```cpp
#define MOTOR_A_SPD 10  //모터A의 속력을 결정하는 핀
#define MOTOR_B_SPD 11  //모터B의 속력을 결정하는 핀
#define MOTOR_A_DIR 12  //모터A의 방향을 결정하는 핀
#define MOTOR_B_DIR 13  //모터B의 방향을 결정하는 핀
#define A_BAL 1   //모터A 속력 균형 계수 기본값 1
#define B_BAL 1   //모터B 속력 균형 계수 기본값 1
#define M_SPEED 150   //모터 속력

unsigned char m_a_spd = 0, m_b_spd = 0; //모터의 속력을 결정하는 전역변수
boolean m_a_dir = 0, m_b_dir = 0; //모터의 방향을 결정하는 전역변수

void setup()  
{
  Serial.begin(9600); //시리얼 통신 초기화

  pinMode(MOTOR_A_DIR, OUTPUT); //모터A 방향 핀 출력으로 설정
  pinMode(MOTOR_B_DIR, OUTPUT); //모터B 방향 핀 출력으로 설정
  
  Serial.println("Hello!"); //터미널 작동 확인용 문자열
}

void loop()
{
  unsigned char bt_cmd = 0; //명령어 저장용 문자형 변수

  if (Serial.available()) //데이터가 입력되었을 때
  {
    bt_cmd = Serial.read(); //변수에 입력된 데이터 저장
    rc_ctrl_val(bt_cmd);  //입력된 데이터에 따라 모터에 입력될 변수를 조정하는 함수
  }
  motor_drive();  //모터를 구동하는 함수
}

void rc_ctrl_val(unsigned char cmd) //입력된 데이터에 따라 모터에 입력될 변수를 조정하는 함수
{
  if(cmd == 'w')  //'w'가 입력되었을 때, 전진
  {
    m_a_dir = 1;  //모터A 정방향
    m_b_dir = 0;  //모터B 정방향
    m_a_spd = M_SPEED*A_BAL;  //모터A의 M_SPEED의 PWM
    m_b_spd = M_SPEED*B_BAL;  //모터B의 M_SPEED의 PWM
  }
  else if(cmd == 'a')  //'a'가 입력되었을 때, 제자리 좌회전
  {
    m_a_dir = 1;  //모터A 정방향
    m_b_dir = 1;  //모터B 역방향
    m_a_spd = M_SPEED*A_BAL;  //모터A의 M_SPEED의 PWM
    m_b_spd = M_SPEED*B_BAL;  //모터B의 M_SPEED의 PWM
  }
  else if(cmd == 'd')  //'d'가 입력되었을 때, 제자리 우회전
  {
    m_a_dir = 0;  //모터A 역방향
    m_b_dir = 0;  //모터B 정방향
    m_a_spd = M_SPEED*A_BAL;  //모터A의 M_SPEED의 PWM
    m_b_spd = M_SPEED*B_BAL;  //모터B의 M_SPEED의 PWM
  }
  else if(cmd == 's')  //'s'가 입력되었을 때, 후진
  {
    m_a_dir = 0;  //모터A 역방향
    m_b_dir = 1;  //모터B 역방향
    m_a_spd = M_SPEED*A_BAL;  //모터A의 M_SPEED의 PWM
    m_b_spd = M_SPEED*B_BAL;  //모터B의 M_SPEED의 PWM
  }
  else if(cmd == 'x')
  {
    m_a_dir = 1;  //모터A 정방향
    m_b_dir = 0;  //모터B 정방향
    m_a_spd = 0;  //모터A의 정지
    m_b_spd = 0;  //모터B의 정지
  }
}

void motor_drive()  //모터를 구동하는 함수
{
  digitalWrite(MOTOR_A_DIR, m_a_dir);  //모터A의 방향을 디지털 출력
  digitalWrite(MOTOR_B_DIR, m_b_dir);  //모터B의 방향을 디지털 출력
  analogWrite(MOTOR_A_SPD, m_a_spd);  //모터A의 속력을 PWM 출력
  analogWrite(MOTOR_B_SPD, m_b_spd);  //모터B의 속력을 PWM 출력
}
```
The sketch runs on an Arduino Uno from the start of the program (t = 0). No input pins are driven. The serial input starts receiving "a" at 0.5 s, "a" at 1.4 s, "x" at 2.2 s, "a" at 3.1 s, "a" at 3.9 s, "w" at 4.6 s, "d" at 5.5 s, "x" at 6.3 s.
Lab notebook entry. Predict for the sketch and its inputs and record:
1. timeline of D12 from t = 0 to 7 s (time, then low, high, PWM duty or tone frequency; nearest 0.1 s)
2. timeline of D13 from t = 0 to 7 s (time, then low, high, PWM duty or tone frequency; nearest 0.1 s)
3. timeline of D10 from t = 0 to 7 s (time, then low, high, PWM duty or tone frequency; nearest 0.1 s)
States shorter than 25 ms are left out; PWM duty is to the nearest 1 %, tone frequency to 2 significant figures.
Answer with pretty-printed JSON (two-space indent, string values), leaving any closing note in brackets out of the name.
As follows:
{
  "timeline of D12 from t = 0 to 7 s": "0 s low; 0.5 s high; 5.5 s low; 6.3 s high",
  "timeline of D13 from t = 0 to 7 s": "0 s low; 0.5 s high; 2.2 s low; 3.1 s high; 4.6 s low",
  "timeline of D10 from t = 0 to 7 s": "0 s low; 0.5 s PWM 59 %; 2.2 s low; 3.1 s PWM 59 %; 6.3 s low"
}
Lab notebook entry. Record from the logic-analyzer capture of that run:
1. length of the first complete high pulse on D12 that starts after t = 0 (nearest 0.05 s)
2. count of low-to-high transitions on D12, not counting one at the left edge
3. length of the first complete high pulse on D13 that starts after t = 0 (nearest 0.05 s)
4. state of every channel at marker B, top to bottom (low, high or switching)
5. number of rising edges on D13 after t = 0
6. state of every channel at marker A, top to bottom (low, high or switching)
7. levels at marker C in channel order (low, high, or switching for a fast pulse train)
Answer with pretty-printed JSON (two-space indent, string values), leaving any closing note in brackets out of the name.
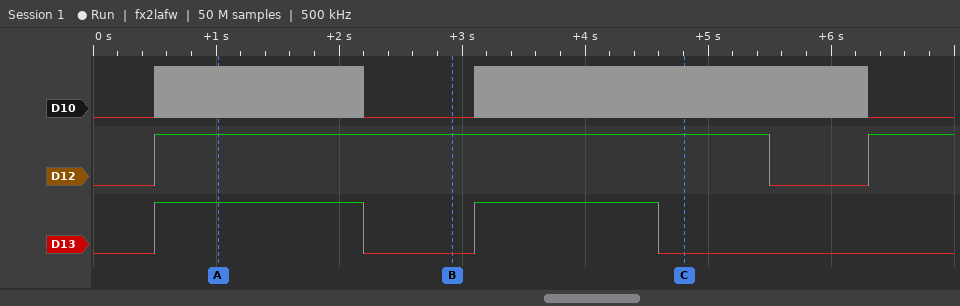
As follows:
{
  "length of the first complete high pulse on D12 that starts after t = 0": "5.00 s",
  "count of low-to-high transitions on D12, not counting one at the left edge": "2",
  "length of the first complete high pulse on D13 that starts after t = 0": "1.70 s",
  "state of every channel at marker B, top to bottom": "D10 low, D12 high, D13 low",
  "number of rising edges on D13 after t = 0": "2",
  "state of every channel at marker A, top to bottom": "D10 switching, D12 high, D13 high",
  "levels at marker C in channel order": "D10 switching, D12 high, D13 low"
}
